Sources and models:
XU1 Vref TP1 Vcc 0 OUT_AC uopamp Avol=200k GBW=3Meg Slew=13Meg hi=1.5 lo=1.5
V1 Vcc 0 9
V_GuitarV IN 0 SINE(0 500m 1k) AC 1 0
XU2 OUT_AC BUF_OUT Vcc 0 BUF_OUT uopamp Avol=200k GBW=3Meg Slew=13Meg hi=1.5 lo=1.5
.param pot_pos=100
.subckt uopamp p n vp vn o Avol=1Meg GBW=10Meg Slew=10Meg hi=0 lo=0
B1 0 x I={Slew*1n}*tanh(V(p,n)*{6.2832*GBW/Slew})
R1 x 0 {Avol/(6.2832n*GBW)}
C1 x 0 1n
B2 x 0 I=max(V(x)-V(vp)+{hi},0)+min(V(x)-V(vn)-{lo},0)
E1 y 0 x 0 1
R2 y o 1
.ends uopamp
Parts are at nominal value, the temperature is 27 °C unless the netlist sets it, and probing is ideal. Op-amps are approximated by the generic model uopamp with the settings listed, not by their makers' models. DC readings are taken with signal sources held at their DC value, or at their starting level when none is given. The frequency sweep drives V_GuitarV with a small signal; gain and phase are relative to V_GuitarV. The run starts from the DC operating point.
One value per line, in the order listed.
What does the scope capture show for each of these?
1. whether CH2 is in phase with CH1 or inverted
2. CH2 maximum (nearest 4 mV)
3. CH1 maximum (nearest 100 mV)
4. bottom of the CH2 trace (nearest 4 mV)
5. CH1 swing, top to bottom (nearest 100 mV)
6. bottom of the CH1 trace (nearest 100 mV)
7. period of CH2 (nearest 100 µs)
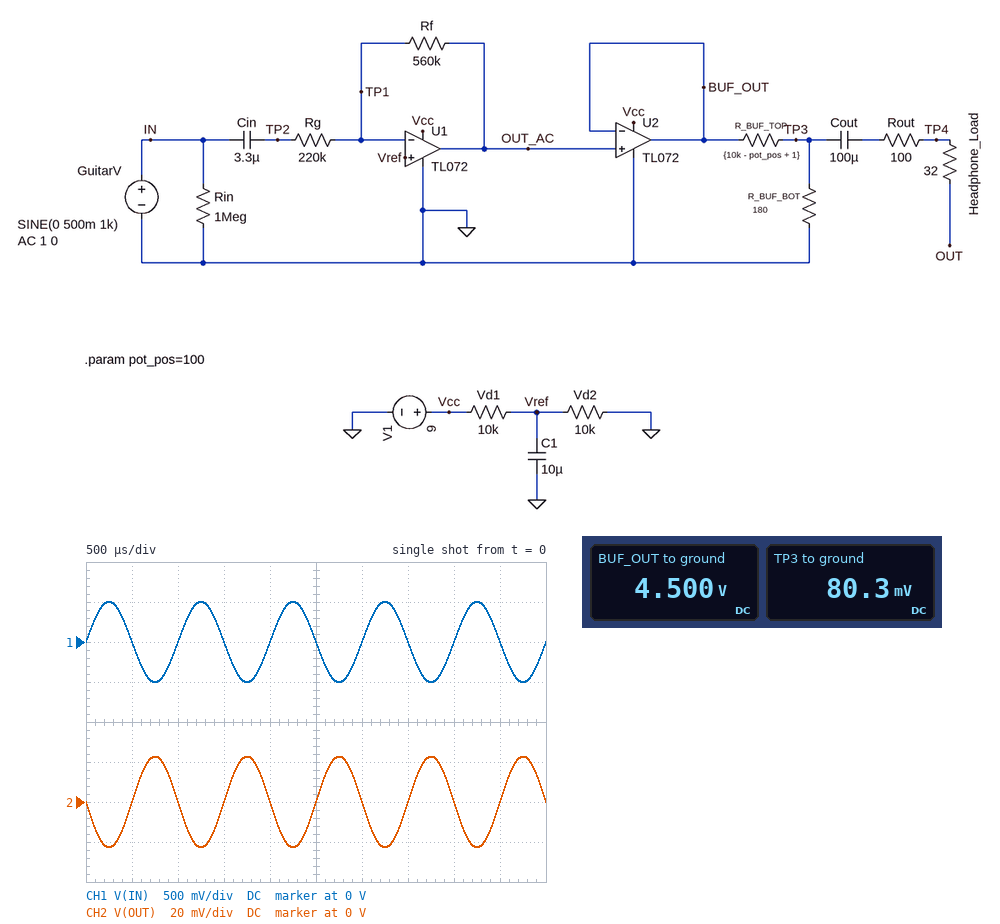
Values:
inverted
24 mV
500 mV
-24 mV
1.0 V
-500 mV
1.0 ms
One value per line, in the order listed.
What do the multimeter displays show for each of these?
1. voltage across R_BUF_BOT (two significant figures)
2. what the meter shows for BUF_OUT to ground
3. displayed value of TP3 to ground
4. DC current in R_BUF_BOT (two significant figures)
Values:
80 mV
4.500 V
80.3 mV
450 µA
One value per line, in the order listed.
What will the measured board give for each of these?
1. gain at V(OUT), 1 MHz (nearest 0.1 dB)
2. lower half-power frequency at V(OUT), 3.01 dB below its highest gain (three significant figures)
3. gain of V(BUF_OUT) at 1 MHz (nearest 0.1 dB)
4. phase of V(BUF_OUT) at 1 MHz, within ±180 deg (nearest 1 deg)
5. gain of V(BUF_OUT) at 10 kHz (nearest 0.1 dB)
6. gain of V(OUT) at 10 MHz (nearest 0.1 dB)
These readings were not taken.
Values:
-31.1 dB
219 mHz
3.9 dB
112 deg
8.1 dB
-59.2 dB
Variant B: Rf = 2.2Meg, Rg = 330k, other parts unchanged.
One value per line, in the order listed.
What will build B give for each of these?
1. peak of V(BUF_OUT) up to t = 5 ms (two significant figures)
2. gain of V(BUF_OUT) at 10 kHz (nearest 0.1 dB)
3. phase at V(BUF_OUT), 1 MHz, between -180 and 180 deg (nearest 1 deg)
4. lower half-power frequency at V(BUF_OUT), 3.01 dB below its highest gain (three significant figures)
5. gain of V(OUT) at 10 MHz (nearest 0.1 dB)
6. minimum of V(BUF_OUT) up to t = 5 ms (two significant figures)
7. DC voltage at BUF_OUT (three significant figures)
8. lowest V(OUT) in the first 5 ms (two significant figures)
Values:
7.5 V
16.5 dB
93 deg
146 mHz
-57.5 dB
1.5 V
4.50 V
-54 mV
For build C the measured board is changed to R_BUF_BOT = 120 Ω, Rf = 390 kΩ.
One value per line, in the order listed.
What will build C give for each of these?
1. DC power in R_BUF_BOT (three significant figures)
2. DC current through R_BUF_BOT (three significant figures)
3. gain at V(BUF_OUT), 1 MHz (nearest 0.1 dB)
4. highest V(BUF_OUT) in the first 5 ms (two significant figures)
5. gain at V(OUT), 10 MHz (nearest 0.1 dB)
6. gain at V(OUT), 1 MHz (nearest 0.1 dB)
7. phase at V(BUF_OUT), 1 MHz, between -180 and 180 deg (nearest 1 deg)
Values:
24.2 µW
449 µA
1.8 dB
5.4 V
-63.7 dB
-36.6 dB
119 deg
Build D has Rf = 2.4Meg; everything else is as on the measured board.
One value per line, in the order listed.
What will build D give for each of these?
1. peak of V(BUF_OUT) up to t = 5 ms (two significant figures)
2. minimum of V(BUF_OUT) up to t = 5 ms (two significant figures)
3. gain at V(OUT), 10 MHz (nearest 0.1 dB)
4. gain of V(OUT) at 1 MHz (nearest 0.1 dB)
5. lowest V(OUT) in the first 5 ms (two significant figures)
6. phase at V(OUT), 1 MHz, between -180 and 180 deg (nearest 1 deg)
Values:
7.5 V
1.5 V
-57.0 dB
-26.9 dB
-54 mV
86 deg
